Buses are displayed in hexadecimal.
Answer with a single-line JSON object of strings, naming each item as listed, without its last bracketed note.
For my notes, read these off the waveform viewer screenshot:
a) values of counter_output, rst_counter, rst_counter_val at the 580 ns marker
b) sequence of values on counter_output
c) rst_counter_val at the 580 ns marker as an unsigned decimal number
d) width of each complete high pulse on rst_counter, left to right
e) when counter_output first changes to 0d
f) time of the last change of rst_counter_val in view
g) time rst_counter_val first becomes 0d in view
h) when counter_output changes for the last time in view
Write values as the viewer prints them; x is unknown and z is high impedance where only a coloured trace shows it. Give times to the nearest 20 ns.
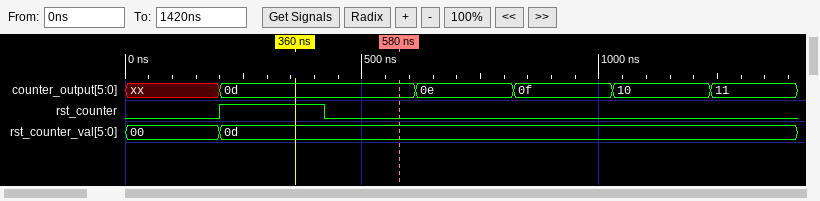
{"values of counter_output, rst_counter, rst_counter_val at the 580 ns marker": "counter_output=0d, rst_counter=0, rst_counter_val=0d", "sequence of values on counter_output": "xx, 0d, 0e, 0f, 10, 11", "rst_counter_val at the 580 ns marker as an unsigned decimal number": "13", "width of each complete high pulse on rst_counter, left to right": "220 ns", "when counter_output first changes to 0d": "200 ns", "time of the last change of rst_counter_val in view": "200 ns", "time rst_counter_val first becomes 0d in view": "200 ns", "when counter_output changes for the last time in view": "1240 ns"}
